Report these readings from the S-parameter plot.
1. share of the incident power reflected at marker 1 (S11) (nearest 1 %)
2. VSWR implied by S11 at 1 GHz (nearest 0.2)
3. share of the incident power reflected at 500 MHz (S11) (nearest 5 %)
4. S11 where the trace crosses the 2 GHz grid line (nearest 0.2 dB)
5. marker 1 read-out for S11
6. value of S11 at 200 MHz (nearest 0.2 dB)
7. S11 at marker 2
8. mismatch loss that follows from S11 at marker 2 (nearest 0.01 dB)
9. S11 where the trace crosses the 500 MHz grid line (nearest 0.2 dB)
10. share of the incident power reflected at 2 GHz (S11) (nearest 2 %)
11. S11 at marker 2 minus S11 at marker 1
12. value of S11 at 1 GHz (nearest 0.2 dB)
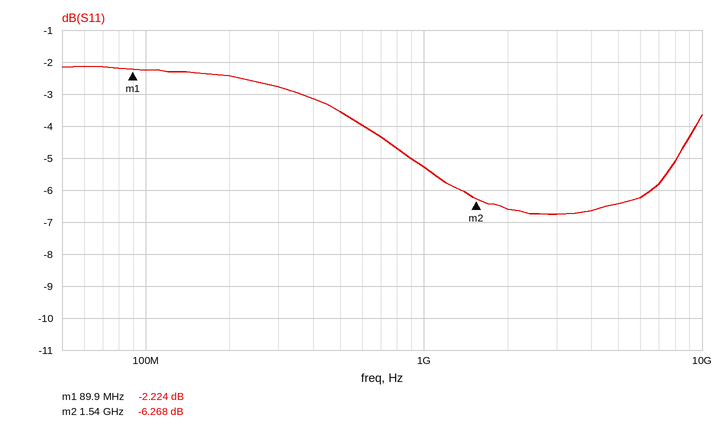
60 %
3.4
45 %
-6.6 dB
-2.224 dB
-2.4 dB
-6.268 dB
1.17 dB
-3.6 dB
22 %
-4.044 dB
-5.2 dB
